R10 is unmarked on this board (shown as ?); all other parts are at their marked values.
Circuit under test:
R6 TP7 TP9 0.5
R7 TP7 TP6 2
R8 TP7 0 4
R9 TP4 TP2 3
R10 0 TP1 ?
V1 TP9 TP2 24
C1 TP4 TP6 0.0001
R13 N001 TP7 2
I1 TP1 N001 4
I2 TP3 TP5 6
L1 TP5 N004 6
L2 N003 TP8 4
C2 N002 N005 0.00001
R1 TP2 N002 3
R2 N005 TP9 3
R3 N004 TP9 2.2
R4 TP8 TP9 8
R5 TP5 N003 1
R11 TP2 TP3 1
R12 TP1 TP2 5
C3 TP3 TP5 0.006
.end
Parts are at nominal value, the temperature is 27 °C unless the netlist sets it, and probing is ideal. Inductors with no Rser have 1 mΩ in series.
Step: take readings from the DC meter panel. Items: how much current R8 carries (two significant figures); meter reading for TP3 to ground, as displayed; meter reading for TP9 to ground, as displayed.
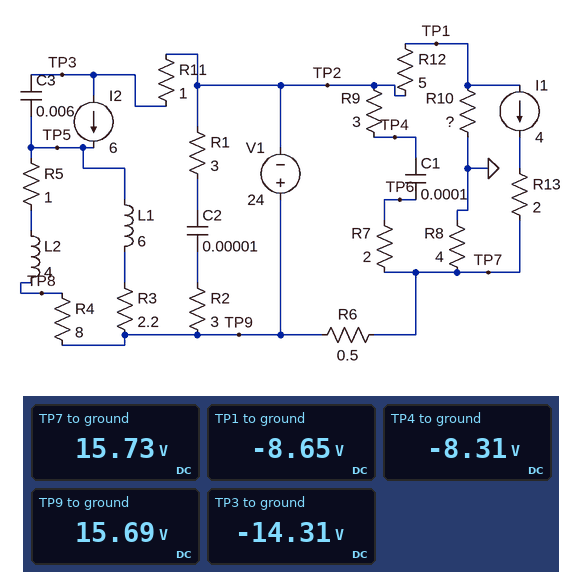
3.9 A
-14.31 V
15.69 V
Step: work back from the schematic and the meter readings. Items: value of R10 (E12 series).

2.2 Ω
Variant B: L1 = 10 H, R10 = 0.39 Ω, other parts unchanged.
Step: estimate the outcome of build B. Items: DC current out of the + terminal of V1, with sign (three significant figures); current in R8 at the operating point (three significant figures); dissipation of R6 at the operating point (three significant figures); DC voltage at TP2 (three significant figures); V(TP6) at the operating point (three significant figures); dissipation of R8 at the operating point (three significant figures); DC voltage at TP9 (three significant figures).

-5.35 A
4.65 A
212 mW
-5.07 V
18.6 V
86.5 W
18.9 V
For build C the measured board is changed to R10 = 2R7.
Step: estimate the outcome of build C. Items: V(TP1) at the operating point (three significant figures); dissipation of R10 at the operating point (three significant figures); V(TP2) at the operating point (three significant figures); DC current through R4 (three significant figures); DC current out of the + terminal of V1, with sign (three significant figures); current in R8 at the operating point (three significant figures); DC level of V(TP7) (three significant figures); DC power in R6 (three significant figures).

-10.2 V
38.4 W
-9.03 V
1.18 A
-6.23 A
3.77 A
15.1 V
26.3 mW
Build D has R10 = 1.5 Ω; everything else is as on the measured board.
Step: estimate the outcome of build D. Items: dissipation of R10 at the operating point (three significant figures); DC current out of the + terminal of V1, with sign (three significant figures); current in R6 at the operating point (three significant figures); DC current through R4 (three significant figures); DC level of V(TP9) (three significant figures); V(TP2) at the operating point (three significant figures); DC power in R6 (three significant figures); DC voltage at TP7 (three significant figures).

26.2 W
-5.82 A
182 mA
1.18 A
16.8 V
-7.18 V
16.5 mW
16.7 V
